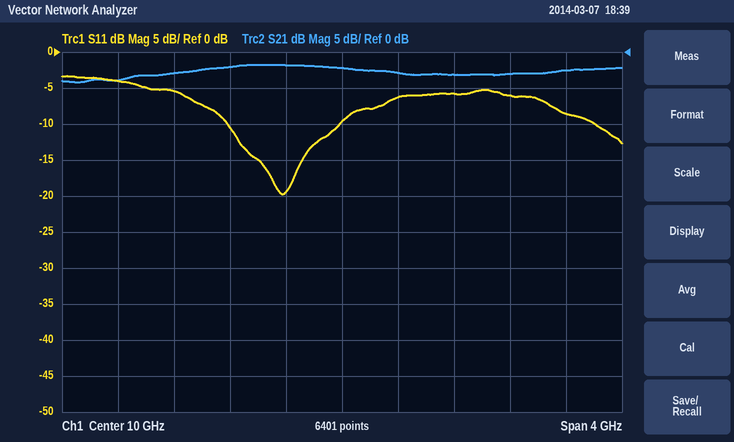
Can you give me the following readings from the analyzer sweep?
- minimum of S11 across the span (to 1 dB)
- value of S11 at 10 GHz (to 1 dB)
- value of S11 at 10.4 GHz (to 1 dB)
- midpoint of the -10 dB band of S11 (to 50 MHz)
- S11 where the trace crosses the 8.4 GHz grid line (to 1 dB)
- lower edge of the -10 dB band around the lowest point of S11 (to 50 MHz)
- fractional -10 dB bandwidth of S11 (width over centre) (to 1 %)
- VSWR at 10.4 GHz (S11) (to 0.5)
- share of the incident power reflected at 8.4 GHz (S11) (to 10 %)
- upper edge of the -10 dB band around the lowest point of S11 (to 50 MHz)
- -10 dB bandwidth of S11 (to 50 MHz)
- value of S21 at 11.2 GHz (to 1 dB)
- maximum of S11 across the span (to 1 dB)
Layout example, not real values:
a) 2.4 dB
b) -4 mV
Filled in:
a) -20 dB
b) -10 dB
c) -6 dB
d) 9.60 GHz
e) -4 dB
f) 9.20 GHz
g) 8 %
h) 3.0
i) 40 %
j) 10.00 GHz
k) 800 MHz
l) -3 dB
m) -3 dB
